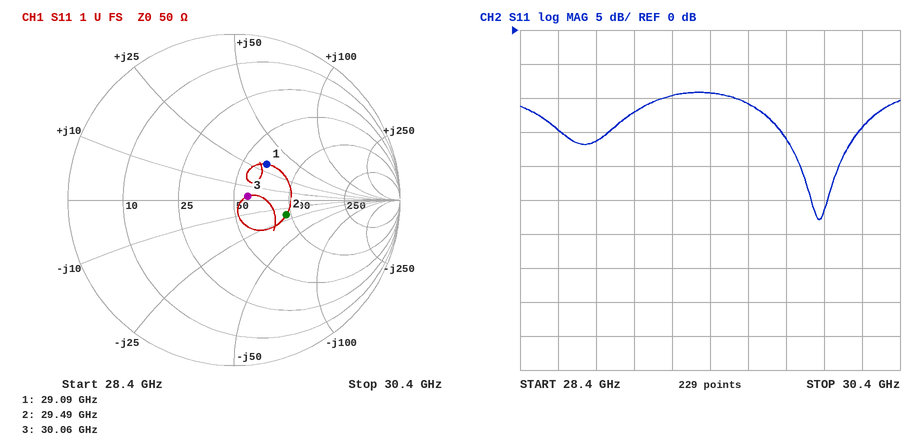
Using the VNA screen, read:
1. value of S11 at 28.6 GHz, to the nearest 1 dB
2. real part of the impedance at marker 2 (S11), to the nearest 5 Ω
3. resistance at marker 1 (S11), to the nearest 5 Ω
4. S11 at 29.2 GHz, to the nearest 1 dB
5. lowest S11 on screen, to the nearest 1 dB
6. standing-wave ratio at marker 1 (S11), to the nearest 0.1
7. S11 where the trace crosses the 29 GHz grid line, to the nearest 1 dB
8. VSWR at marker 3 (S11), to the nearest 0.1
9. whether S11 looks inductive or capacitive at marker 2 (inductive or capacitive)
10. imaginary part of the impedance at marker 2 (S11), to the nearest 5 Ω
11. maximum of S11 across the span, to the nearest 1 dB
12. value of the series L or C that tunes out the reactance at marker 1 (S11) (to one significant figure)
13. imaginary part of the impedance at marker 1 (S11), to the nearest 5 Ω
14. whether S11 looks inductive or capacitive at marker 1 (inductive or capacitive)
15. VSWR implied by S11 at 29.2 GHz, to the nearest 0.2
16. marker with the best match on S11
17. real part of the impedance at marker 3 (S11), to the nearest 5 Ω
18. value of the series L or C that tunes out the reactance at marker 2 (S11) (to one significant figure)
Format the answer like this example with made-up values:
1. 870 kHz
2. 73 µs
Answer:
1. -15 dB
2. 95 Ω
3. 65 Ω
4. -10 dB
5. -28 dB
6. 1.8
7. -12 dB
8. 1.2
9. capacitive
10. -20 Ω
11. -9 dB
12. 200 fF
13. +30 Ω
14. inductive
15. 2.0
16. marker 3
17. 60 Ω
18. 100 pH
